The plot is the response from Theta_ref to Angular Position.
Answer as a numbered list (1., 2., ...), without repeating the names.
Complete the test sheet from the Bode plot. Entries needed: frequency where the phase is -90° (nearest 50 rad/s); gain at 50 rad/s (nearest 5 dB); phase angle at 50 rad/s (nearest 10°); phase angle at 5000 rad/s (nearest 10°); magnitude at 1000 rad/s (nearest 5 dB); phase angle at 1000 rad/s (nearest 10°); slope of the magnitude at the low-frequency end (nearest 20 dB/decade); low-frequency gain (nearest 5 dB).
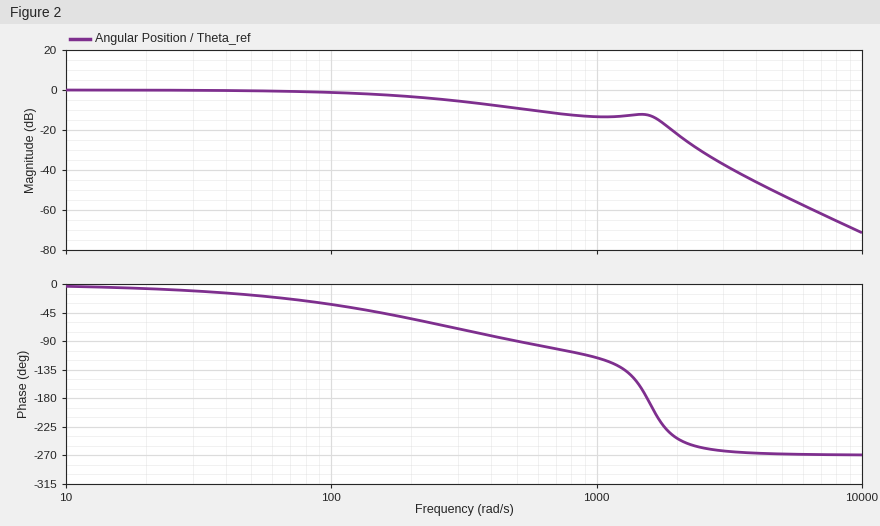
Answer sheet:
1. 500 rad/s
2. 0 dB
3. -20°
4. -270°
5. -15 dB
6. -120°
7. 0 dB/decade
8. 0 dB
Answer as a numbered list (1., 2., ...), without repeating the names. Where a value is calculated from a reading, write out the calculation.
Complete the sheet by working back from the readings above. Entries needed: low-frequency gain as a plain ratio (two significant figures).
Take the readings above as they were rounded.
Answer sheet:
1. 10^(0 / 20) = 1.0
